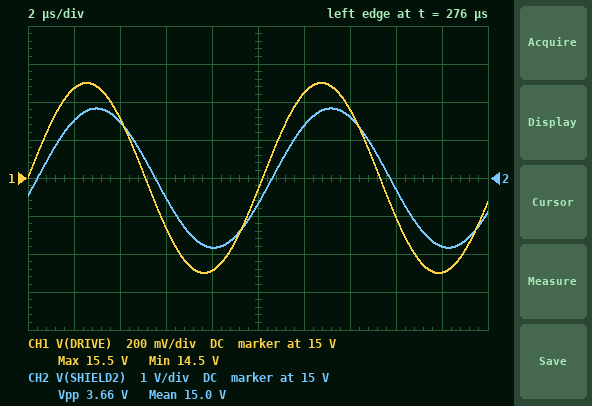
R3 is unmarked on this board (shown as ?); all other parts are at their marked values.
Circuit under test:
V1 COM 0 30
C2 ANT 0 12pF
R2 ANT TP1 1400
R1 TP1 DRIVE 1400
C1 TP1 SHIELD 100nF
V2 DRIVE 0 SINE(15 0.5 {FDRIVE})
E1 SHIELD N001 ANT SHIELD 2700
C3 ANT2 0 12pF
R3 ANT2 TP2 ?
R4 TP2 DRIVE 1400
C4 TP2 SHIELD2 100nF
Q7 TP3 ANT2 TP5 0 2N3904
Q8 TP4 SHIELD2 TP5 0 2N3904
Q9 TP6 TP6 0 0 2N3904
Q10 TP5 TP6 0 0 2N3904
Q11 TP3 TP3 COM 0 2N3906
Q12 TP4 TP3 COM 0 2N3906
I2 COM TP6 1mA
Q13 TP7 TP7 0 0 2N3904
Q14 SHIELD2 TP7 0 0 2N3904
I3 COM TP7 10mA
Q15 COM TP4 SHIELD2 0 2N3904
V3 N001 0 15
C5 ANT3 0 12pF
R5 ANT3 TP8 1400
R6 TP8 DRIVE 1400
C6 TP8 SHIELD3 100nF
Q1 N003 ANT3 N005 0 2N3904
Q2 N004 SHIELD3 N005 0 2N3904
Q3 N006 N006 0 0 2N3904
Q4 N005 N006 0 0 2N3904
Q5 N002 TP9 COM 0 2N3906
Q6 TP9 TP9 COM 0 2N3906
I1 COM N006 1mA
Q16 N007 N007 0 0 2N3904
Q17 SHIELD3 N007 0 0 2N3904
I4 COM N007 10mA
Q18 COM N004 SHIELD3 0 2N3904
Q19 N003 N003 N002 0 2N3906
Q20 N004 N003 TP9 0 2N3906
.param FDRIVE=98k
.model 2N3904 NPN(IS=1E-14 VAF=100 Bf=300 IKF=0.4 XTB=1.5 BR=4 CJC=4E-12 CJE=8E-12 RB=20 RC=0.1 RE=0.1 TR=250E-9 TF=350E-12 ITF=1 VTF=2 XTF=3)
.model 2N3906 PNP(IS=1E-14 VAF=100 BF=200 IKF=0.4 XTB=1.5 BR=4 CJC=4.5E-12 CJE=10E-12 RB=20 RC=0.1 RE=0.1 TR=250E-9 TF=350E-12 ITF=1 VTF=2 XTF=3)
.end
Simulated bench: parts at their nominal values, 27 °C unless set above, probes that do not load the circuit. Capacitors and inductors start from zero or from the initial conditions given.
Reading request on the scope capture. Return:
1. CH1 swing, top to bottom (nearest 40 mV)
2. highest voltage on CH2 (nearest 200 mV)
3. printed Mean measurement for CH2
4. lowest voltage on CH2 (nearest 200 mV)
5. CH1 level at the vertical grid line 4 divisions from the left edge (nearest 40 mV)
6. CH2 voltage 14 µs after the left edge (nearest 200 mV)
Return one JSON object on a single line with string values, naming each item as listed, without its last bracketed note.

{"CH1 swing, top to bottom": "1.00 V", "highest voltage on CH2": "16.8 V", "printed Mean measurement for CH2": "15.0 V", "lowest voltage on CH2": "13.2 V", "CH1 level at the vertical grid line 4 divisions from the left edge": "14.52 V", "CH2 voltage 14 µs after the left edge": "16.6 V"}
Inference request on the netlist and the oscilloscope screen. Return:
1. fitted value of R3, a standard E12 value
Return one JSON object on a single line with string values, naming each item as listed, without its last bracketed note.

{"fitted value of R3, a standard E12 value": "1 kΩ"}
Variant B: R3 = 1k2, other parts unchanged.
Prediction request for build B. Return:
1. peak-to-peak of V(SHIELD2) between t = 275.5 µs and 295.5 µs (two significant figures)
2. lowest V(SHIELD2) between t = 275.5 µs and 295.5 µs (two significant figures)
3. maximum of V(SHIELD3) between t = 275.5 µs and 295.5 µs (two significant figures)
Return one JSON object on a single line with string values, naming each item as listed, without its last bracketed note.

{"peak-to-peak of V(SHIELD2) between t = 275.5 µs and 295.5 µs": "7.1 V", "lowest V(SHIELD2) between t = 275.5 µs and 295.5 µs": "11 V", "maximum of V(SHIELD3) between t = 275.5 µs and 295.5 µs": "23 V"}
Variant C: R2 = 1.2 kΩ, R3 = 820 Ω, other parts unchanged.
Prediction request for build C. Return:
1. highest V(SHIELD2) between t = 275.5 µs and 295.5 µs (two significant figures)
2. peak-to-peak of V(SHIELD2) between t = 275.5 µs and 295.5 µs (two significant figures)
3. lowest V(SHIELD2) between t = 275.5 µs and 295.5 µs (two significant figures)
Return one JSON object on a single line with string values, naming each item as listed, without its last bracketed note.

{"highest V(SHIELD2) between t = 275.5 µs and 295.5 µs": "16 V", "peak-to-peak of V(SHIELD2) between t = 275.5 µs and 295.5 µs": "2.5 V", "lowest V(SHIELD2) between t = 275.5 µs and 295.5 µs": "14 V"}
